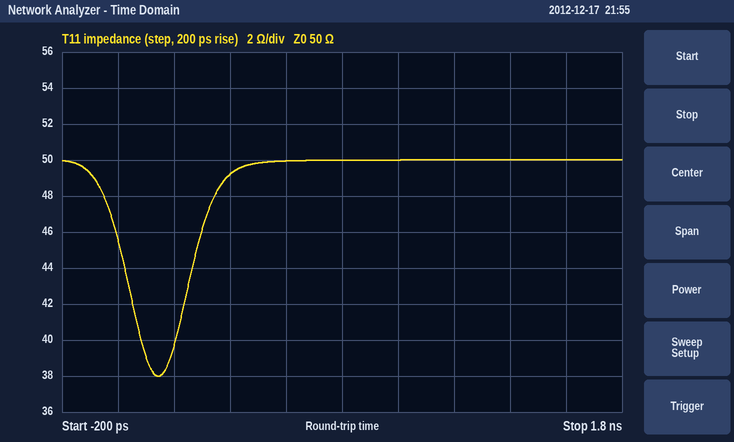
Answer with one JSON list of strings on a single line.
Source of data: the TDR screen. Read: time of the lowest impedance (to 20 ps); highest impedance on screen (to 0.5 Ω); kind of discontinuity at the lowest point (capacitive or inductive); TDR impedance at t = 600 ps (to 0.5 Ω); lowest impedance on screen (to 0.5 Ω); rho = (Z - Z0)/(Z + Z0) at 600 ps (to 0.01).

["140 ps", "50.0 Ω", "capacitive", "50.0 Ω", "38.0 Ω", "0.00"]
